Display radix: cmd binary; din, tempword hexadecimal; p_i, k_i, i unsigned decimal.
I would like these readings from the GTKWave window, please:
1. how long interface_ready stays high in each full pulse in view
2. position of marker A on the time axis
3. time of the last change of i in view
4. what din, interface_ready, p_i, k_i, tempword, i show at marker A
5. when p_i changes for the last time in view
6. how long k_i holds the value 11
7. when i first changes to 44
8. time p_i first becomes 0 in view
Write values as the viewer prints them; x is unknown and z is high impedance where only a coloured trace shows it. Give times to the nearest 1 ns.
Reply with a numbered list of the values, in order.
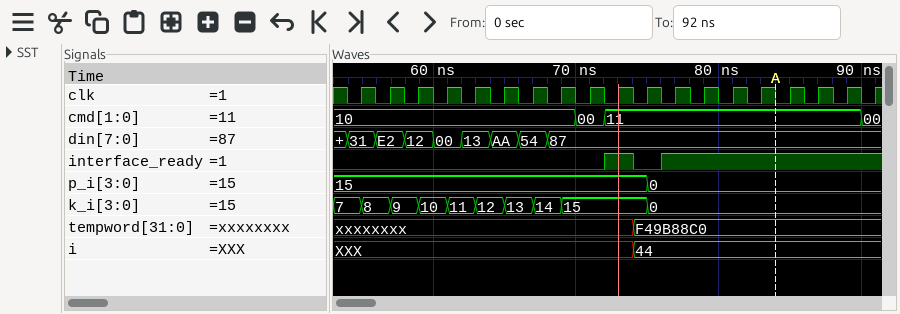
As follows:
1. 2 ns
2. 84 ns
3. 74 ns
4. din=87, interface_ready=1, p_i=0, k_i=0, tempword=F49B88C0, i=44
5. 75 ns
6. 2 ns
7. 74 ns
8. 75 ns
